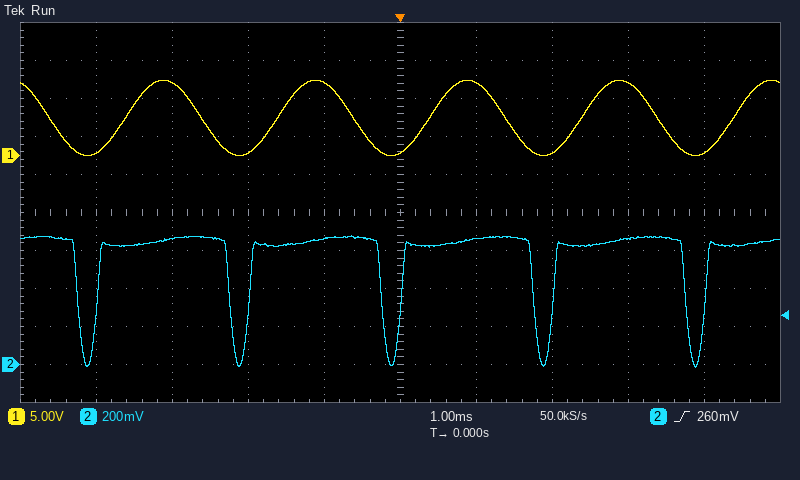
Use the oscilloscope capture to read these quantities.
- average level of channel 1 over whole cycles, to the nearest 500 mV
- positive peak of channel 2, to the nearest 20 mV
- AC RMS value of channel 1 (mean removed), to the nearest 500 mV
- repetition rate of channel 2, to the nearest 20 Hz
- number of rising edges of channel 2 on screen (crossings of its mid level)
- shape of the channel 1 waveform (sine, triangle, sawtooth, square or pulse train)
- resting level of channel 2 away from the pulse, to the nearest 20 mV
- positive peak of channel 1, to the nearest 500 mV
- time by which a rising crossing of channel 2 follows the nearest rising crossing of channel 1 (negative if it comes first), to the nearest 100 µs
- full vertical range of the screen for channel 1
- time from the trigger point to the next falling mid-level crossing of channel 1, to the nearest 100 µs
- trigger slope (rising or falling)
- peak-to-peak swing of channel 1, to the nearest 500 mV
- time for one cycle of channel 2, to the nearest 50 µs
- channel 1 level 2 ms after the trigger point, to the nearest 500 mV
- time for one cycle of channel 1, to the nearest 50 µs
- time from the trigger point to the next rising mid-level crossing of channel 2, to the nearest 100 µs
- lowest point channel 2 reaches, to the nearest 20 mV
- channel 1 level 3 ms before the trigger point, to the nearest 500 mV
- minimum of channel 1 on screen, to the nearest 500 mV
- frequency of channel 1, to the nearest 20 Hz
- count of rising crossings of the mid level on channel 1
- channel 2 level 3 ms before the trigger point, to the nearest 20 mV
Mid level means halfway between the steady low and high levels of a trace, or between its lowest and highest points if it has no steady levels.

5.0 V
680 mV
3.5 V
500 Hz
5
sine
640 mV
10.0 V
-400 µs
50 V
1.4 ms
rising
10.0 V
2.00 ms
500 mV
2.00 ms
2.0 ms
-20 mV
9.5 V
0.0 V
500 Hz
5
660 mV
